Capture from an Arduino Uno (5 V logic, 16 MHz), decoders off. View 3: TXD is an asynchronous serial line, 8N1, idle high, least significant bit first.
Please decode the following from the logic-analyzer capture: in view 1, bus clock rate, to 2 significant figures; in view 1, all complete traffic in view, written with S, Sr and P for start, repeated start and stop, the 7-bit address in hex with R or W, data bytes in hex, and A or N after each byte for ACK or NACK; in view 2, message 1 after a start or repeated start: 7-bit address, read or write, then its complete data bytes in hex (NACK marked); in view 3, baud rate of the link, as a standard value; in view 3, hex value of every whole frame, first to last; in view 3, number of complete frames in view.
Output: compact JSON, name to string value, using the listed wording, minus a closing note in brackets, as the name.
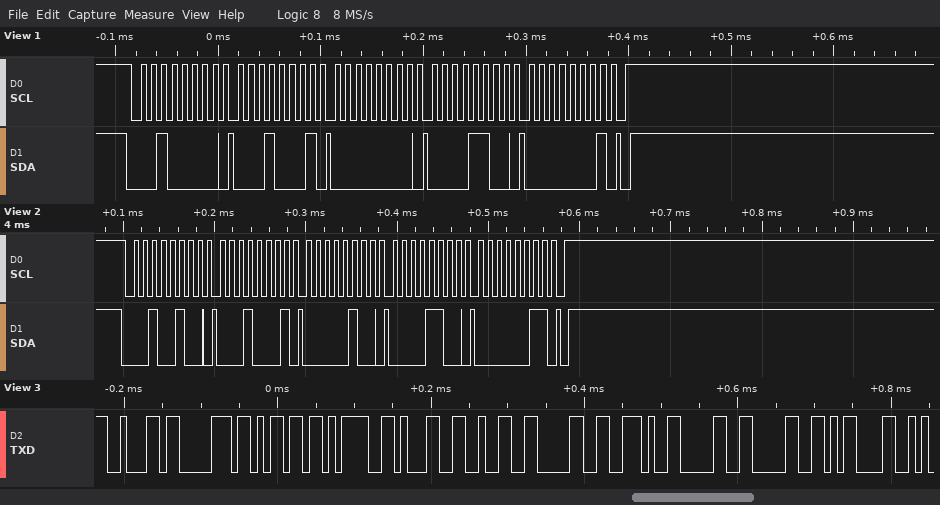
{"in view 1, bus clock rate, to 2 significant figures": "100 kHz", "in view 1, all complete traffic in view, written with S, Sr and P for start, repeated start and stop, the 7-bit address in hex with R or W, data bytes in hex, and A or N after each byte for ACK or NACK": "S 10W A 11 A 00 A 0C A 01 A P", "in view 2, message 1 after a start or repeated start: 7-bit address, read or write, then its complete data bytes in hex": "0x12 write: 11 04 0C 03", "in view 3, baud rate of the link, as a standard value": "115200 baud", "in view 3, hex value of every whole frame, first to last": "62 70 6D 3D 31 32 30 2E 30 30 0D", "in view 3, number of complete frames in view": "11"}
